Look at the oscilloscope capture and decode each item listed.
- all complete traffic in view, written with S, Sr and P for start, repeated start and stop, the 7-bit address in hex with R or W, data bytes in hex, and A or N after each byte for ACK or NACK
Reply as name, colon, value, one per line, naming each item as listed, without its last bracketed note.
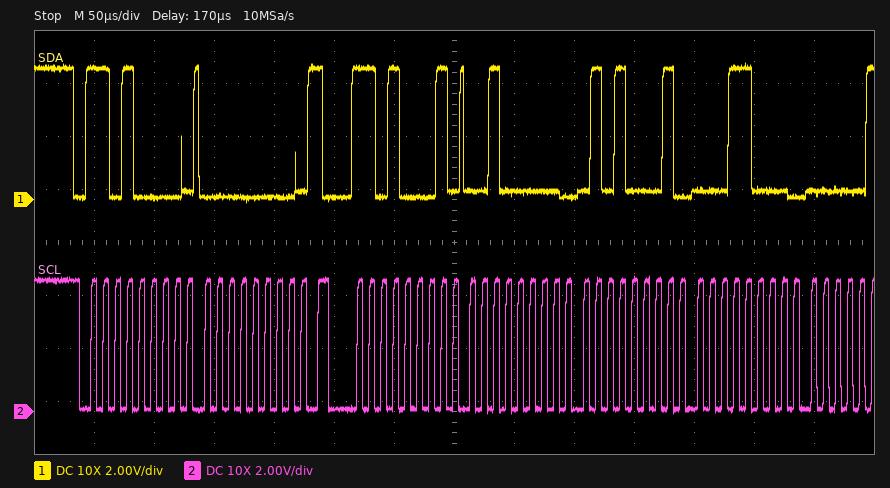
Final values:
all complete traffic in view, written with S, Sr and P for start, repeated start and stop, the 7-bit address in hex with R or W, data bytes in hex, and A or N after each byte for ACK or NACK: S 68W A 00 A Sr 68R A 20 A 51 A 18 A
